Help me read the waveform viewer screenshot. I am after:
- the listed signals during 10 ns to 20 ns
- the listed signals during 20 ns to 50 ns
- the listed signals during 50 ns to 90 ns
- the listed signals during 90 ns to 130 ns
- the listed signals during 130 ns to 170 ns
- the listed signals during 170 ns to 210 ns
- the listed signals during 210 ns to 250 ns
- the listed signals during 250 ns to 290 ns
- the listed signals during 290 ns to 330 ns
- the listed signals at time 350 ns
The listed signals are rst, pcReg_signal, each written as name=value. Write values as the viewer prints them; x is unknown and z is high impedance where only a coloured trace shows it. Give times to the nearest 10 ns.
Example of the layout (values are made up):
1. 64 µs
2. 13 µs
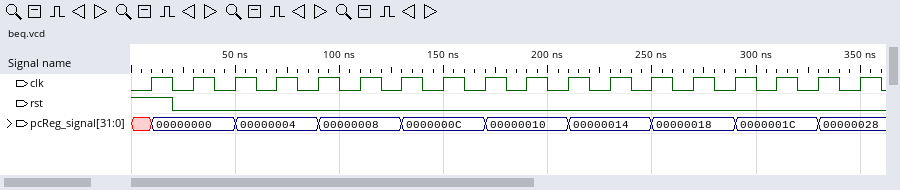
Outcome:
1. rst=1, pcReg_signal=00000000
2. rst=0, pcReg_signal=00000000
3. rst=0, pcReg_signal=00000004
4. rst=0, pcReg_signal=00000008
5. rst=0, pcReg_signal=0000000C
6. rst=0, pcReg_signal=00000010
7. rst=0, pcReg_signal=00000014
8. rst=0, pcReg_signal=00000018
9. rst=0, pcReg_signal=0000001C
10. rst=0, pcReg_signal=00000028
